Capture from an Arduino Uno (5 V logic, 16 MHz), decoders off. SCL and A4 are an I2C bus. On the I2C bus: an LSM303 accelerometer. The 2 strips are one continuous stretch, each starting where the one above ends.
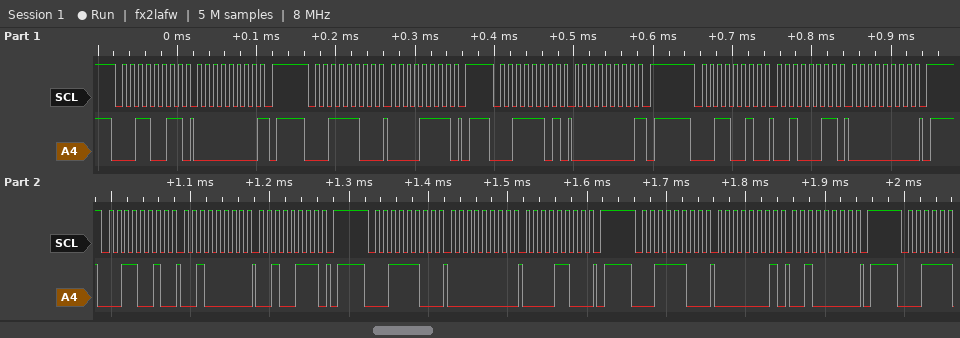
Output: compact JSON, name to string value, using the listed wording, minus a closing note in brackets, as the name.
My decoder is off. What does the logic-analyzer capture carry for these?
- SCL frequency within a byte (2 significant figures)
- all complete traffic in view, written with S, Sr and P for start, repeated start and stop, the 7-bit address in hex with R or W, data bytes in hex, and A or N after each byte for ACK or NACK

{"SCL frequency within a byte": "100 kHz", "all complete traffic in view, written with S, Sr and P for start, repeated start and stop, the 7-bit address in hex with R or W, data bytes in hex, and A or N after each byte for ACK or NACK": "S 19R A 00 N P S 1EW A 0F A P S 1ER A 00 N P S 19W A 23 A 00 A P S 19W A 20 A 27 A P S 1EW A 00 A 0C A P S 1EW A 01 A 20 A P"}
